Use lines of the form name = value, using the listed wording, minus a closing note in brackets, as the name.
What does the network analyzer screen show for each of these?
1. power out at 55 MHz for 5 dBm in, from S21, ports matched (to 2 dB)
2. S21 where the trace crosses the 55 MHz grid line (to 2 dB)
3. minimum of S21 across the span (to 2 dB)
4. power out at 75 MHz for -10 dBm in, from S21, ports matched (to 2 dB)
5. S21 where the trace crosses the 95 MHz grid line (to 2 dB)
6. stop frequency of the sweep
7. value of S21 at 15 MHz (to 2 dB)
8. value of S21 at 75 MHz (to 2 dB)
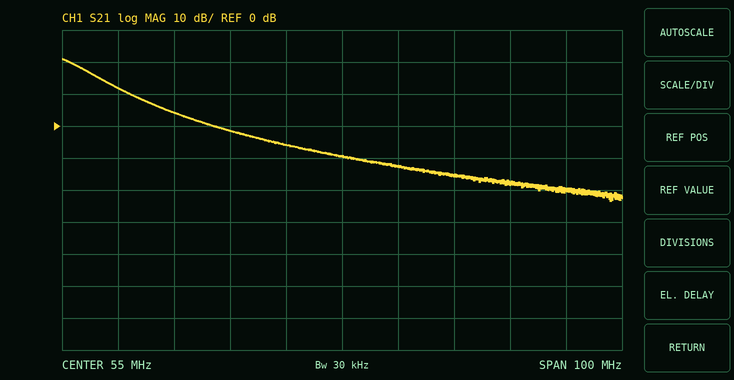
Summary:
power out at 55 MHz for 5 dBm in, from S21, ports matched = -4 dBm
S21 where the trace crosses the 55 MHz grid line = -10 dB
minimum of S21 across the span = -24 dB
power out at 75 MHz for -10 dBm in, from S21, ports matched = -26 dBm
S21 where the trace crosses the 95 MHz grid line = -20 dB
stop frequency of the sweep = 105 MHz
value of S21 at 15 MHz = 12 dB
value of S21 at 75 MHz = -16 dB
